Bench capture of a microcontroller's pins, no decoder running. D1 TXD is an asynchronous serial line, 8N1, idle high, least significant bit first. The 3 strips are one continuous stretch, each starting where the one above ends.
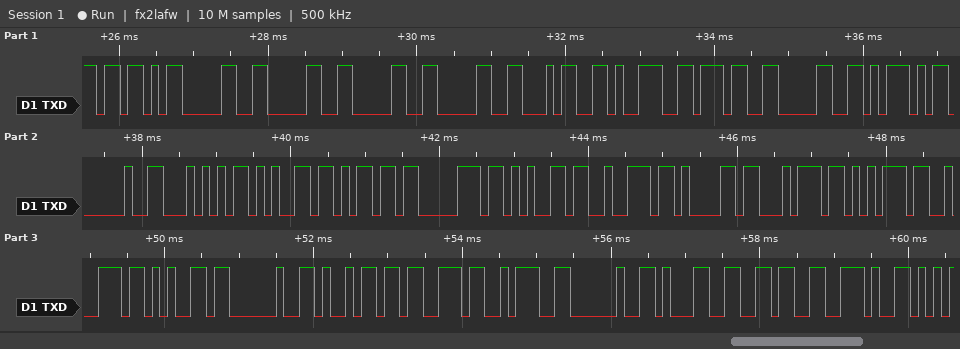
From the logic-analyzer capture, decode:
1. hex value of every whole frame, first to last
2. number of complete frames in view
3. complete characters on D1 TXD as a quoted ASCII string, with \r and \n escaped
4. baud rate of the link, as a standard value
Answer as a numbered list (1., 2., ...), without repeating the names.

1. 0x5B 0x30 0x30 0x30 0x30 0x34 0x39 0x37 0x30 0x5D 0x20 0x54 0x65 0x6D 0x70 0x65 0x72 0x61 0x74 0x75 0x72 0x65 0x20 0x69 0x73 0x3A 0x20 0x31 0x36 0x2E
2. 30
3. "[00004970] Temperature is: 16."
4. 9600 baud
